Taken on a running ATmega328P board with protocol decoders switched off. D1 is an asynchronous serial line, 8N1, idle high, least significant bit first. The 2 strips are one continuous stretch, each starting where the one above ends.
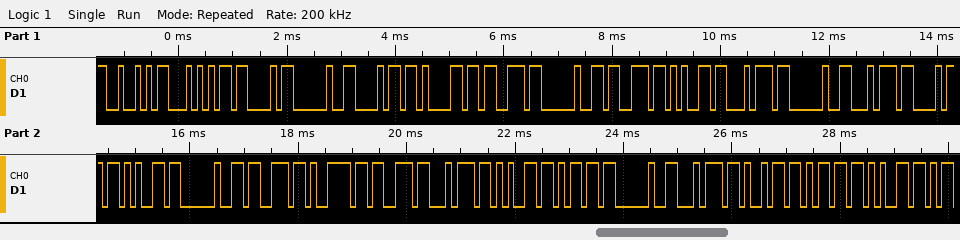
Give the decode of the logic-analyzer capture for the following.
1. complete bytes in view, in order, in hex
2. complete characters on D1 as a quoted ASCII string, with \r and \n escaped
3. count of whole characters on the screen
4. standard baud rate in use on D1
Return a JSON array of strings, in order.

["52 54 43 20 68 61 73 20 73 65 74 20 74 68 65 20 73 79 73 74 65 6D 20 74 69 6D 65", "\"RTC has set the system time\"", "27", "9600 baud"]
